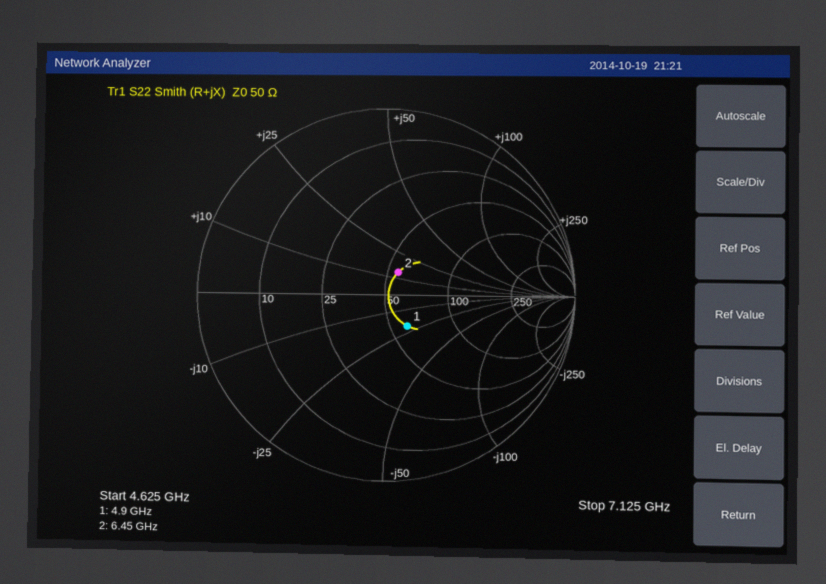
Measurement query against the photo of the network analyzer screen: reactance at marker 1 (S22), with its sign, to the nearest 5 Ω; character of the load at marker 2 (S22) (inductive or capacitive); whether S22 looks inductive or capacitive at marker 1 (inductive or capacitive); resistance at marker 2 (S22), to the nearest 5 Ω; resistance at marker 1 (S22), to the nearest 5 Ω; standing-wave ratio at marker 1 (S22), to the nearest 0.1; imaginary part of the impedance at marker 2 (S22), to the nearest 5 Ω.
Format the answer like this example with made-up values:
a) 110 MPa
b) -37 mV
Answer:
a) -20 Ω
b) inductive
c) capacitive
d) 55 Ω
e) 60 Ω
f) 1.5
g) +15 Ω
